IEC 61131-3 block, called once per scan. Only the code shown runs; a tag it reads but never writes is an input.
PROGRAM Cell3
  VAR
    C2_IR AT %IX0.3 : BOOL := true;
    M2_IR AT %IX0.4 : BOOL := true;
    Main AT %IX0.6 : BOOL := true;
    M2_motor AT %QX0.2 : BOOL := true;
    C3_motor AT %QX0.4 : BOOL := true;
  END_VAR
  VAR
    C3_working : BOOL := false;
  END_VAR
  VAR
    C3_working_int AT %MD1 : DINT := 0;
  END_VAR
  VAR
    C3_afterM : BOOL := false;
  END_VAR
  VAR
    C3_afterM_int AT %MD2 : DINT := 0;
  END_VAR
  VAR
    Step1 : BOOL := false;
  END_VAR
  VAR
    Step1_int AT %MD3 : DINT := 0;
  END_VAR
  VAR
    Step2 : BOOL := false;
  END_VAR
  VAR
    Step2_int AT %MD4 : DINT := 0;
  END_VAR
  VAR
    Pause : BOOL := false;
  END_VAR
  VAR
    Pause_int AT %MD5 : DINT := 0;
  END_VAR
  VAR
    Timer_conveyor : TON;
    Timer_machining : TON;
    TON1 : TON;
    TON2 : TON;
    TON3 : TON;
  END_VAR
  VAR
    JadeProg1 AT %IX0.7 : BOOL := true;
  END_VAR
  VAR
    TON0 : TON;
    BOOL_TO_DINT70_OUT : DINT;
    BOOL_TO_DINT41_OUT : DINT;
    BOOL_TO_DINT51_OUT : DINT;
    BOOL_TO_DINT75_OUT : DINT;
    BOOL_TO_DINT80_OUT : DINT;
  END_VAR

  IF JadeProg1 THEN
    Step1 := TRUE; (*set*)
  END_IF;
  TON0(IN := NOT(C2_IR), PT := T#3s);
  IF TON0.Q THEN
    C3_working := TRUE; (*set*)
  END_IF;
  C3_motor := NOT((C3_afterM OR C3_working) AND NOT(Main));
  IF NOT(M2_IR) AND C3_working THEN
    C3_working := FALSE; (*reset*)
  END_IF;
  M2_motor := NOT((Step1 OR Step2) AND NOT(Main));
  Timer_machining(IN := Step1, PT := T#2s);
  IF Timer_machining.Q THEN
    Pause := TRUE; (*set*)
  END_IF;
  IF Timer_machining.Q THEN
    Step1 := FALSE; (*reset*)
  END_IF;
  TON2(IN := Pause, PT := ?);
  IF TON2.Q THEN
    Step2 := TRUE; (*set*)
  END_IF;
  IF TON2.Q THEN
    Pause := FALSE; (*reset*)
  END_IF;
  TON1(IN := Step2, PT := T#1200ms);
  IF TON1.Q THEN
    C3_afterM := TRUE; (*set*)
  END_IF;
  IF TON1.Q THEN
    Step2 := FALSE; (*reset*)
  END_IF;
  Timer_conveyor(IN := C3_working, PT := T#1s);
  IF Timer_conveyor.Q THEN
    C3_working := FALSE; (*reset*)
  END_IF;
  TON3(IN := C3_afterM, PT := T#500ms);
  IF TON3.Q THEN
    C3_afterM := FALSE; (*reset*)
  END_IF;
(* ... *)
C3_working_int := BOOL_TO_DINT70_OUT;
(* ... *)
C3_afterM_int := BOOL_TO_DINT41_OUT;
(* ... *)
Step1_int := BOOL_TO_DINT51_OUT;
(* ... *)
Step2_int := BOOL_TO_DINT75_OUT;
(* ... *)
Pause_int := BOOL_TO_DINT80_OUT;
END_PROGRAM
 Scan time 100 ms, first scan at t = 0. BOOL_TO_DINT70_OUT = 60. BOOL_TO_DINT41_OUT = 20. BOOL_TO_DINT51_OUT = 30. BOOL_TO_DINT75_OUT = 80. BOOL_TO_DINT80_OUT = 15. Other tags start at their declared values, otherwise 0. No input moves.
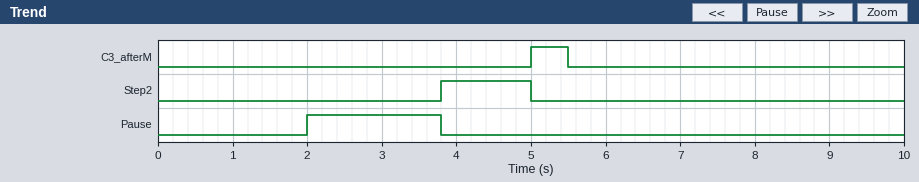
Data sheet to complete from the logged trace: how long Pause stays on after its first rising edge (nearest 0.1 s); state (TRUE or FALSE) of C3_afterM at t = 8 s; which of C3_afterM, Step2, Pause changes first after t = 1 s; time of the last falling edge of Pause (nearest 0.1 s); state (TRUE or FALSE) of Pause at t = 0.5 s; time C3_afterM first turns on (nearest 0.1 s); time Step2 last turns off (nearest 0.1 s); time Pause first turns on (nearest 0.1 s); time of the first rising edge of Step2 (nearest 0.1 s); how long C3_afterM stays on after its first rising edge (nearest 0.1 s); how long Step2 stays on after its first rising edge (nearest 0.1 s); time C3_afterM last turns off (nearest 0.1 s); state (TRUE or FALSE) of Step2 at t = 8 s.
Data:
1.8 s
FALSE
Pause
3.8 s
FALSE
5.0 s
5.0 s
2.0 s
3.8 s
0.5 s
1.2 s
5.5 s
FALSE
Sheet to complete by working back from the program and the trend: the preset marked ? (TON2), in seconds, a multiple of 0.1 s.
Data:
1.8 s
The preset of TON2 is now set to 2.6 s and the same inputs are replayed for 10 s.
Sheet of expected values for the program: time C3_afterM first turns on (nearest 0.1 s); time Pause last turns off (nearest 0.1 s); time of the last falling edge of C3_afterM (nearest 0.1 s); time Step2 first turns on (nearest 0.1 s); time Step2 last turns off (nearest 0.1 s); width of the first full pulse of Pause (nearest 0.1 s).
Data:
5.8 s
4.6 s
6.3 s
4.6 s
5.8 s
2.6 s
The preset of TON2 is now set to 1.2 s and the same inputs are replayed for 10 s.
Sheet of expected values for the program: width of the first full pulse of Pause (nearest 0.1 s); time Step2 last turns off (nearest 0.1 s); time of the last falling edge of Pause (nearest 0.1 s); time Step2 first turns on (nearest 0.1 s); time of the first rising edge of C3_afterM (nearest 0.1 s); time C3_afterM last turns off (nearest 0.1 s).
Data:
1.2 s
4.4 s
3.2 s
3.2 s
4.4 s
4.9 s
